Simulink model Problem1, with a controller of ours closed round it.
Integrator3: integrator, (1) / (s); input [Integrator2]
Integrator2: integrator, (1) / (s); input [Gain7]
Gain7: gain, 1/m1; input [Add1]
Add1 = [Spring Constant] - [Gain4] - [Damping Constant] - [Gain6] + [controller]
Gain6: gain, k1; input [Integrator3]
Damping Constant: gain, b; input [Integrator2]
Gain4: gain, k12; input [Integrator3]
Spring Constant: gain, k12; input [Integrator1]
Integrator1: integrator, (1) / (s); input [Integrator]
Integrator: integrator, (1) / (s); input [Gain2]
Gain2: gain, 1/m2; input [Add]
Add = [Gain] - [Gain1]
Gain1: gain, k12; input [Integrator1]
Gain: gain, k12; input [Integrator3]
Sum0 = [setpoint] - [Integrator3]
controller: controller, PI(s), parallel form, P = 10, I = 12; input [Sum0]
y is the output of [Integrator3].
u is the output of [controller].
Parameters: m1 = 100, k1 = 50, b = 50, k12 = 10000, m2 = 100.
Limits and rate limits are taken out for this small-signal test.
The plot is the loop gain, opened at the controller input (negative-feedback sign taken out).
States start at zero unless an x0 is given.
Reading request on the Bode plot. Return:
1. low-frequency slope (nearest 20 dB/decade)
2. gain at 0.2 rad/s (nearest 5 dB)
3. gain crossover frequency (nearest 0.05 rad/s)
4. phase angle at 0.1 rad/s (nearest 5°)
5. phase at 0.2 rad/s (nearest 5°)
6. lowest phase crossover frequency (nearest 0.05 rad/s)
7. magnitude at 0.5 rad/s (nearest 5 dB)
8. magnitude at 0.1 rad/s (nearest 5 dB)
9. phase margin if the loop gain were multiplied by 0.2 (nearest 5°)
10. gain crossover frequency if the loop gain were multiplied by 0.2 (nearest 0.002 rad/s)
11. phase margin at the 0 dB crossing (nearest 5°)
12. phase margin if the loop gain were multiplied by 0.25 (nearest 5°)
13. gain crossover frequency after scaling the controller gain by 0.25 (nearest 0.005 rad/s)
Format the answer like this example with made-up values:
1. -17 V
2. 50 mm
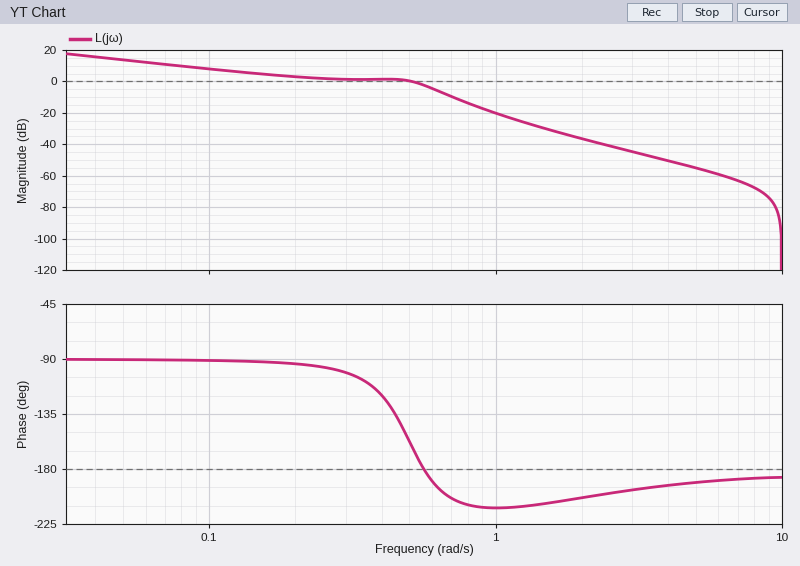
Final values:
1. -20 dB/decade
2. 5 dB
3. 0.50 rad/s
4. -90°
5. -95°
6. 0.55 rad/s
7. 0 dB
8. 10 dB
9. 90°
10. 0.048 rad/s
11. 20°
12. 90°
13. 0.060 rad/s
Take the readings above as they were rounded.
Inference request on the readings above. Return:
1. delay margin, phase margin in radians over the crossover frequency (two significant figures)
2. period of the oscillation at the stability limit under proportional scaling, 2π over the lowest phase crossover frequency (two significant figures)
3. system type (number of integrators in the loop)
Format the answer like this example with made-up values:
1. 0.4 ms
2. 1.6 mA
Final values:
1. 0.70 s
2. 11 s
3. 1
